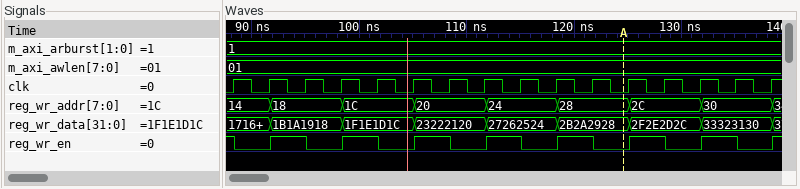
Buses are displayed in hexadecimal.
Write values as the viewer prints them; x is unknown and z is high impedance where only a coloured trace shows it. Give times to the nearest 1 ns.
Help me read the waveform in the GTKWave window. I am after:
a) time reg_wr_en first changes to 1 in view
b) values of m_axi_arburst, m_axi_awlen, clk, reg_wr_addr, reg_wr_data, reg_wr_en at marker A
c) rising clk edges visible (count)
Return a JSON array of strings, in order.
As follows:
["92 ns", "m_axi_arburst=1, m_axi_awlen=01, clk=0, reg_wr_addr=28, reg_wr_data=2B2A2928, reg_wr_en=0", "16"]
